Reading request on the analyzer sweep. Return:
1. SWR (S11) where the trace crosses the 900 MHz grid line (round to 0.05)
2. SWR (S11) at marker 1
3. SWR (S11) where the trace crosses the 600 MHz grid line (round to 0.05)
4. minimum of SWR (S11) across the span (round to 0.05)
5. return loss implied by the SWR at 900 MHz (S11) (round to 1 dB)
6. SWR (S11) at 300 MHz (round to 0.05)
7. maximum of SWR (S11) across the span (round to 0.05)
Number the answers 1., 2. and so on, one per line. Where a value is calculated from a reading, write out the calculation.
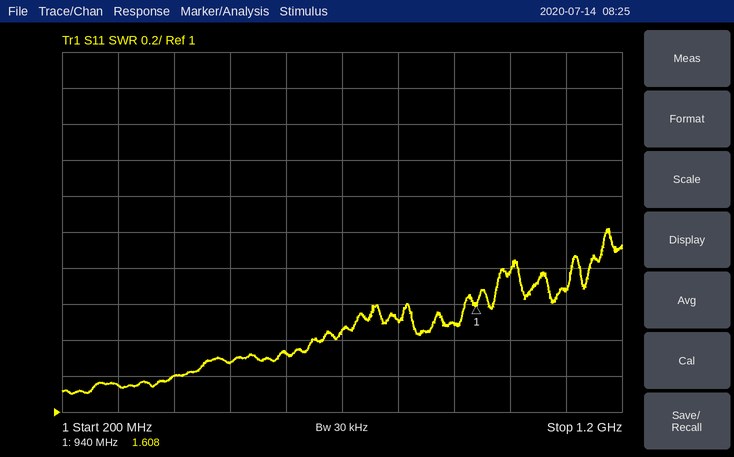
1. 1.50
2. 1.608
3. 1.35
4. 1.10
5. −20 log10((1.5 − 1)/(1.5 + 1)) ≈ 14 dB
6. 1.15
7. 2.00
